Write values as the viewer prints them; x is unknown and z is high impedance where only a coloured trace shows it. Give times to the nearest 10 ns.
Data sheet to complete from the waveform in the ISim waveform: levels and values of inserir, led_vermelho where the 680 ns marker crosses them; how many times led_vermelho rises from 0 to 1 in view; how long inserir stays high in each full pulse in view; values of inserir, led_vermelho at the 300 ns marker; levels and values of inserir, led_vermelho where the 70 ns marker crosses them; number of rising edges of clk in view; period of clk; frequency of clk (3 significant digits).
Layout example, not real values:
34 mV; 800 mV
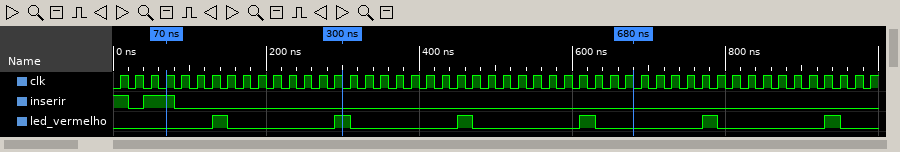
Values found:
inserir=0, led_vermelho=0; 6; 40 ns; inserir=0, led_vermelho=1; inserir=1, led_vermelho=0; 50; 20 ns; 50.0 MHz
